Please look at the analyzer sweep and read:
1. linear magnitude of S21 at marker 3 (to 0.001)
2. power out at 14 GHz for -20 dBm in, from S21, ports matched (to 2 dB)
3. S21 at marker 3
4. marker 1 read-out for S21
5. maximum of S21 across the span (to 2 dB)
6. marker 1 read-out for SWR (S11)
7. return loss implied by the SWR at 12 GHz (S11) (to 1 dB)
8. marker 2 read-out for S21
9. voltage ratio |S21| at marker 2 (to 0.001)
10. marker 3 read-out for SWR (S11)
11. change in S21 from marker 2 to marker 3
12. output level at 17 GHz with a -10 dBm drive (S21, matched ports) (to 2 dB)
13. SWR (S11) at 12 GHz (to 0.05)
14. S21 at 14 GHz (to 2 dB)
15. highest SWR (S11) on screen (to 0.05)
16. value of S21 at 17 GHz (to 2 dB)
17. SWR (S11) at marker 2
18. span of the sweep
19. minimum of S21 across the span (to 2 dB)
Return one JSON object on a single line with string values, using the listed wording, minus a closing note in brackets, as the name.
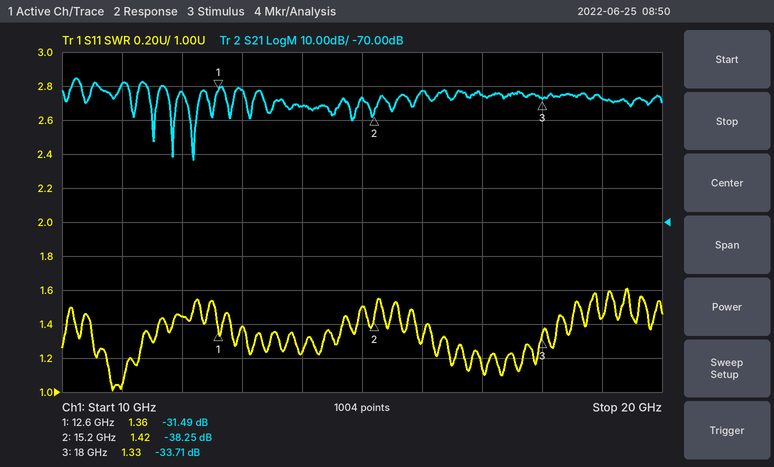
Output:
{"linear magnitude of S21 at marker 3": "0.021", "power out at 14 GHz for -20 dBm in, from S21, ports matched": "-56 dBm", "S21 at marker 3": "-33.71 dB", "marker 1 read-out for S21": "-31.49 dB", "maximum of S21 across the span": "-28 dB", "marker 1 read-out for SWR": "1.36", "return loss implied by the SWR at 12 GHz (S11)": "15 dB", "marker 2 read-out for S21": "-38.25 dB", "voltage ratio |S21| at marker 2": "0.012", "marker 3 read-out for SWR": "1.33", "change in S21 from marker 2 to marker 3": "4.54 dB", "output level at 17 GHz with a -10 dBm drive (S21, matched ports)": "-42 dBm", "SWR (S11) at 12 GHz": "1.45", "S21 at 14 GHz": "-36 dB", "highest SWR (S11) on screen": "1.60", "value of S21 at 17 GHz": "-32 dB", "SWR (S11) at marker 2": "1.42", "span of the sweep": "10 GHz", "minimum of S21 across the span": "-52 dB"}
